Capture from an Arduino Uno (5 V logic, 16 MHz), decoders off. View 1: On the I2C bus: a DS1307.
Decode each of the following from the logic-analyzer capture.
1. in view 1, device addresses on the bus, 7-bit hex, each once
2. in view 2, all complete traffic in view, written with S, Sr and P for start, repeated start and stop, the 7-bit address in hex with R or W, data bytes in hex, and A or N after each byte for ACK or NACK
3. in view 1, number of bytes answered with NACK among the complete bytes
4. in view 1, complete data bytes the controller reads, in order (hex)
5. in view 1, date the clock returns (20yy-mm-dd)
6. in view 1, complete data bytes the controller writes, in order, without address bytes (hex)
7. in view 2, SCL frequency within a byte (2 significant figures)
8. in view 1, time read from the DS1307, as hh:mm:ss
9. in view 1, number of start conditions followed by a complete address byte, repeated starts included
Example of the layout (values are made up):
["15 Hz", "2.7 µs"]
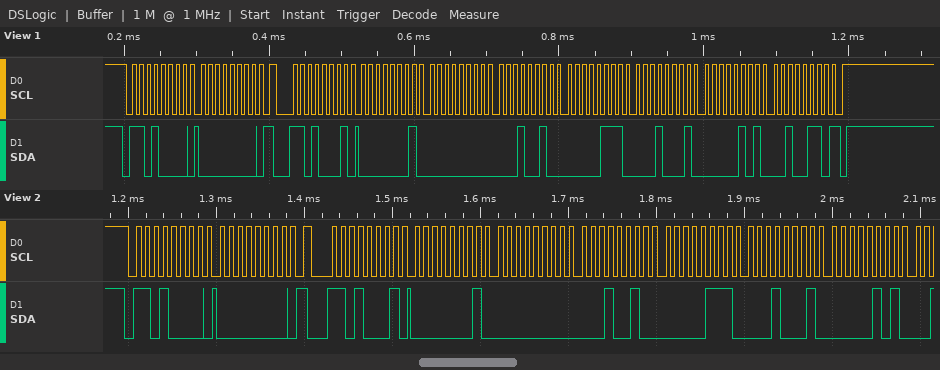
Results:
["0x68", "S 68W A 00 A Sr 68R A 01 A 00 A 12 A 07 A 11 A 05 A", "1", "01 00 12 07 11 05 26", "2026-05-11", "00", "100 kHz", "12:00:01", "2"]
